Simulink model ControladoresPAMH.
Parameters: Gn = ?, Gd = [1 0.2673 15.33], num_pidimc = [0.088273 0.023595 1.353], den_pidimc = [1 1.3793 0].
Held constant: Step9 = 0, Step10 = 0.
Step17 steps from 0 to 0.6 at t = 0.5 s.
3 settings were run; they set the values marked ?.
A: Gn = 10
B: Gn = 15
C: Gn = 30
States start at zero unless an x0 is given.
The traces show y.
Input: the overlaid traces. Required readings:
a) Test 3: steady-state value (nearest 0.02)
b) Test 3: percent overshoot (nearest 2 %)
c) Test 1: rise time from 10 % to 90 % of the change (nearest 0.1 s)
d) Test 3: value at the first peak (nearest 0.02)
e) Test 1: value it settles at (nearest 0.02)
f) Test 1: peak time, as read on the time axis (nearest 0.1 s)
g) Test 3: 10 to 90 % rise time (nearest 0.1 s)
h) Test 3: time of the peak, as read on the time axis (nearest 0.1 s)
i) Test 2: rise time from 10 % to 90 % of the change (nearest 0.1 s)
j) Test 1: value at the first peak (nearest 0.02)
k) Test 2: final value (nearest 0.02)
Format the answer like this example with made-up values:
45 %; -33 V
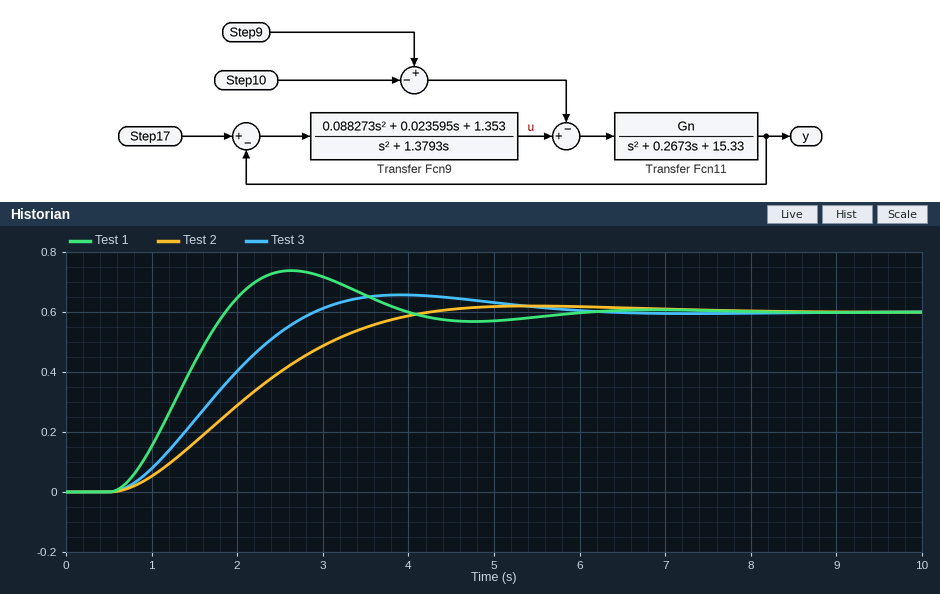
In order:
0.60; 10 %; 0.9 s; 0.66; 0.60; 2.6 s; 1.6 s; 3.9 s; 2.4 s; 0.74; 0.60
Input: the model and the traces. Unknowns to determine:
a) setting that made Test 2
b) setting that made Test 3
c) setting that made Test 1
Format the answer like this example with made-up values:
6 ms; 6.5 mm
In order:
A; B; C
